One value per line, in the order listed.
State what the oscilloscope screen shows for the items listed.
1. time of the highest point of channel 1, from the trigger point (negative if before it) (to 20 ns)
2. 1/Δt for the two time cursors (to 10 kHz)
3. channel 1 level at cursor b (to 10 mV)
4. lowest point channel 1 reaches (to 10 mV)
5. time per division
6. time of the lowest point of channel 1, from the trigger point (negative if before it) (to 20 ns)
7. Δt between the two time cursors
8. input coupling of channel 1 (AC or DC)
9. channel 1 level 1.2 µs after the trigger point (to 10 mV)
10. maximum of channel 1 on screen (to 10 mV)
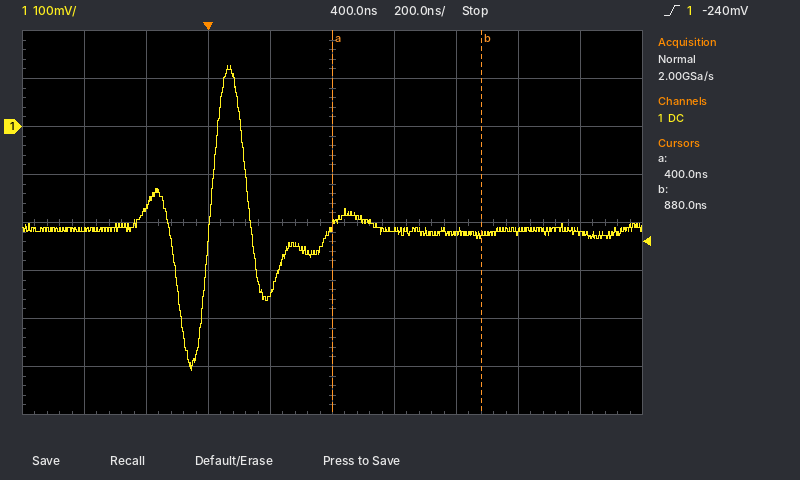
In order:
+60 ns
2.08 MHz
-230 mV
-510 mV
200 ns
-60 ns
480 ns
DC
-220 mV
130 mV
